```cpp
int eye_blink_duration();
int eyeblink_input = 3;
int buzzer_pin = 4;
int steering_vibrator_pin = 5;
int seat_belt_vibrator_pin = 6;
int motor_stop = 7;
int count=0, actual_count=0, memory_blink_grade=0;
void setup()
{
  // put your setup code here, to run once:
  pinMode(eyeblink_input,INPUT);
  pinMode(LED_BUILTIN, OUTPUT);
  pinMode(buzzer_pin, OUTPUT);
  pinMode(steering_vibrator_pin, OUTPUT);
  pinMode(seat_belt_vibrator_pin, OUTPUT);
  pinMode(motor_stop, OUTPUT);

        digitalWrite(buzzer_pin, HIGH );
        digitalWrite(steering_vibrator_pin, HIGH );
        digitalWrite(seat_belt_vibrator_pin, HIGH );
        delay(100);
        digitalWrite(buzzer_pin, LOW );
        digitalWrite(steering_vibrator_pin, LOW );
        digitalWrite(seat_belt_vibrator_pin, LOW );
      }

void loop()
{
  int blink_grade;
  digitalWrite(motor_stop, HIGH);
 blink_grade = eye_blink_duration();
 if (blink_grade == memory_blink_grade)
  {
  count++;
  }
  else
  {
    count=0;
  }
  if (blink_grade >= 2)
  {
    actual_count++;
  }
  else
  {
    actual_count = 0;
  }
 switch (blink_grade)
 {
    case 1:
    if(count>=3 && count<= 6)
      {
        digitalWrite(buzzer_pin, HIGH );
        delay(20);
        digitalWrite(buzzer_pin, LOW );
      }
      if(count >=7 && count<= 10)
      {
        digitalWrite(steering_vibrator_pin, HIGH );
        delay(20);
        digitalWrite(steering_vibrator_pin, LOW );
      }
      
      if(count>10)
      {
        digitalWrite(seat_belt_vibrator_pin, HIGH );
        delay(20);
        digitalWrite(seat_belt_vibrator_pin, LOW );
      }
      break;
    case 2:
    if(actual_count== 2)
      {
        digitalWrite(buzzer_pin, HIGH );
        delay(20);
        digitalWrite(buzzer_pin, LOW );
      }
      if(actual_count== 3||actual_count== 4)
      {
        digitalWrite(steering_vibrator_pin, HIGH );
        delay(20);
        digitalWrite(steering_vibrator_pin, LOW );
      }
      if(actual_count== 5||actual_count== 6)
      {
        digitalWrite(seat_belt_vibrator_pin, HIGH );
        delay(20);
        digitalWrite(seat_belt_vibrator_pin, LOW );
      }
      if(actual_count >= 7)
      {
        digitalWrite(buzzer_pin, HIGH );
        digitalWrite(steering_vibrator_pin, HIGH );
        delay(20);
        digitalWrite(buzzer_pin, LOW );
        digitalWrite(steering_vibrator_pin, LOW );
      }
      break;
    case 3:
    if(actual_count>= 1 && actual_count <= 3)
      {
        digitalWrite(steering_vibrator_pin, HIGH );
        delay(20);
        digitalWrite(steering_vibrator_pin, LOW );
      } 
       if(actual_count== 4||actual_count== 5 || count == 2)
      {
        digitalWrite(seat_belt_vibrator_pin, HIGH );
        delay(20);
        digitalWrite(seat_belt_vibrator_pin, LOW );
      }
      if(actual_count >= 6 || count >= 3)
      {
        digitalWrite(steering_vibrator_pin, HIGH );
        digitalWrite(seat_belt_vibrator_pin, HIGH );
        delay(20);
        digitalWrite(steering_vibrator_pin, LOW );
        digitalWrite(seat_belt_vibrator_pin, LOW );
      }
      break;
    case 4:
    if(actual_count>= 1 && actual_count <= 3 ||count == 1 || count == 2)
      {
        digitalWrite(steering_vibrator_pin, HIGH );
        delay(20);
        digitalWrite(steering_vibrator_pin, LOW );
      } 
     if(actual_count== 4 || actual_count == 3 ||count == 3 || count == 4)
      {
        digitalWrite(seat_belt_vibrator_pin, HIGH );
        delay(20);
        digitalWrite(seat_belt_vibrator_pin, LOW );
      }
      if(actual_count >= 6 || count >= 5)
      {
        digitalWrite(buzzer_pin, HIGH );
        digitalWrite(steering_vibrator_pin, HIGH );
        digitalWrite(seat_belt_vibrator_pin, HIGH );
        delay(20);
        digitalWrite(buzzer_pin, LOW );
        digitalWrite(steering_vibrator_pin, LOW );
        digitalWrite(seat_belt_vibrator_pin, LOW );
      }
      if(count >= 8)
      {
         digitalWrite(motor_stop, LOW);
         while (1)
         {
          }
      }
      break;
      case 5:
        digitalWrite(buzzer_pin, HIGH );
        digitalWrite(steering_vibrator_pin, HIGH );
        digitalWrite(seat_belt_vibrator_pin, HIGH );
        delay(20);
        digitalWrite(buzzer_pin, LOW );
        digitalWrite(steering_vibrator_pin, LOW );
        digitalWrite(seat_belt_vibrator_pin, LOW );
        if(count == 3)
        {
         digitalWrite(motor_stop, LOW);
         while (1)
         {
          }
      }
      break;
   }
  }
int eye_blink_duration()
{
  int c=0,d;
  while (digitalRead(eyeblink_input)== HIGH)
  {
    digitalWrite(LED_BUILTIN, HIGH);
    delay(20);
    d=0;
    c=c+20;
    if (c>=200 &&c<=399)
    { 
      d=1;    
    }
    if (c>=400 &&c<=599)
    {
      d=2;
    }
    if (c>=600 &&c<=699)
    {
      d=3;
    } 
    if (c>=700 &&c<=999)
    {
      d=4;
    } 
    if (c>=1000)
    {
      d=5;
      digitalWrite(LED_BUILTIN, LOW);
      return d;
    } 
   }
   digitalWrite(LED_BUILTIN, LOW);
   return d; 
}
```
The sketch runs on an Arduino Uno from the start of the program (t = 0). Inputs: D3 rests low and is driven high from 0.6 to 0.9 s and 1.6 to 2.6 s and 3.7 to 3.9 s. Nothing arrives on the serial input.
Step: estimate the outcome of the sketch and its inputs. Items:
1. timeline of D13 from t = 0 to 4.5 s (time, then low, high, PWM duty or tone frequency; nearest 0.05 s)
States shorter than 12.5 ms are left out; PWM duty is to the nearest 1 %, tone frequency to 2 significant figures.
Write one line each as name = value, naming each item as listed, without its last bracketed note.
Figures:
timeline of D13 from t = 0 to 4.5 s = 0 s low; 0.6 s high; 0.9 s low; 1.6 s high; 2.6 s low; 3.7 s high; 3.9 s low
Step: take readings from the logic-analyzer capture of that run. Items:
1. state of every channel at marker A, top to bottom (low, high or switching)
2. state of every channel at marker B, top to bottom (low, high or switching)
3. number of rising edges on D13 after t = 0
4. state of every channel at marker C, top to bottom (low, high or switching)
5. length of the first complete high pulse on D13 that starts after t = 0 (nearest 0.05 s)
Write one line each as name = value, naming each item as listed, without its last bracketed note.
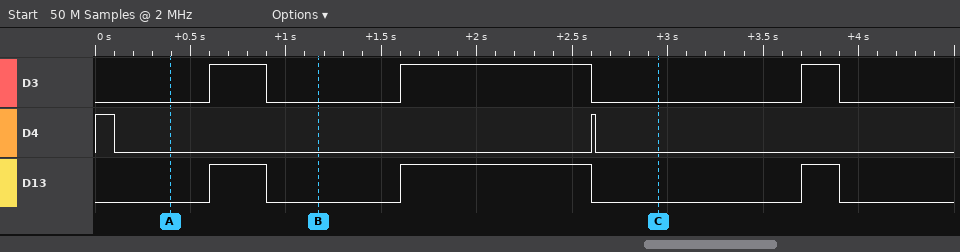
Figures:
state of every channel at marker A, top to bottom = D3 low, D4 low, D13 low
state of every channel at marker B, top to bottom = D3 low, D4 low, D13 low
number of rising edges on D13 after t = 0 = 3
state of every channel at marker C, top to bottom = D3 low, D4 low, D13 low
length of the first complete high pulse on D13 that starts after t = 0 = 0.30 s
